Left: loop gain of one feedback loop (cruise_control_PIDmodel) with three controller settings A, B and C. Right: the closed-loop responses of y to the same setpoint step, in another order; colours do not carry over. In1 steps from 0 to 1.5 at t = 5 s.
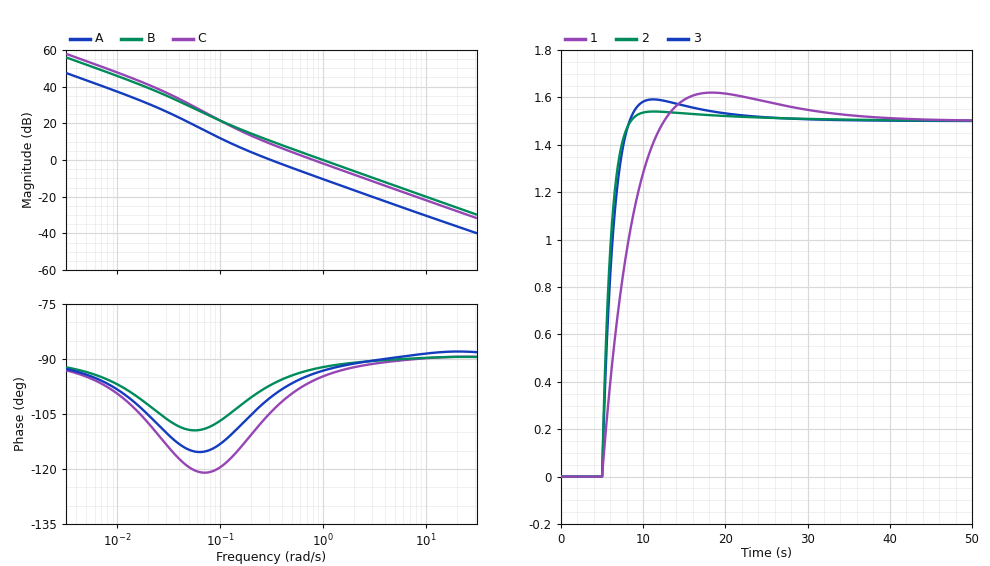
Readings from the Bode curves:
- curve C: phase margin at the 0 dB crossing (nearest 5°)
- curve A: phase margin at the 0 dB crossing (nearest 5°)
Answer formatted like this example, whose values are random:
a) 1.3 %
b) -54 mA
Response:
a) 85°
b) 80°
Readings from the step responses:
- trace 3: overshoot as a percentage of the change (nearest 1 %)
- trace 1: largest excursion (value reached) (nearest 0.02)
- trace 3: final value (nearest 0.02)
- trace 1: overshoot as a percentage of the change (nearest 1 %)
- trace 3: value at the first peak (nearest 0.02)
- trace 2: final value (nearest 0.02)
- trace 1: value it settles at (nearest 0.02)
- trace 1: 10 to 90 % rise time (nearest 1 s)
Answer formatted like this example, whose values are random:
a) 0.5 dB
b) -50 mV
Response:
a) 6 %
b) 1.62
c) 1.50
d) 8 %
e) 1.60
f) 1.50
g) 1.50
h) 5 s
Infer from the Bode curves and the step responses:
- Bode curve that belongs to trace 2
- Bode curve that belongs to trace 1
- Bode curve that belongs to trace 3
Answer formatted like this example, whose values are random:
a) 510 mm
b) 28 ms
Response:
a) B
b) A
c) C
